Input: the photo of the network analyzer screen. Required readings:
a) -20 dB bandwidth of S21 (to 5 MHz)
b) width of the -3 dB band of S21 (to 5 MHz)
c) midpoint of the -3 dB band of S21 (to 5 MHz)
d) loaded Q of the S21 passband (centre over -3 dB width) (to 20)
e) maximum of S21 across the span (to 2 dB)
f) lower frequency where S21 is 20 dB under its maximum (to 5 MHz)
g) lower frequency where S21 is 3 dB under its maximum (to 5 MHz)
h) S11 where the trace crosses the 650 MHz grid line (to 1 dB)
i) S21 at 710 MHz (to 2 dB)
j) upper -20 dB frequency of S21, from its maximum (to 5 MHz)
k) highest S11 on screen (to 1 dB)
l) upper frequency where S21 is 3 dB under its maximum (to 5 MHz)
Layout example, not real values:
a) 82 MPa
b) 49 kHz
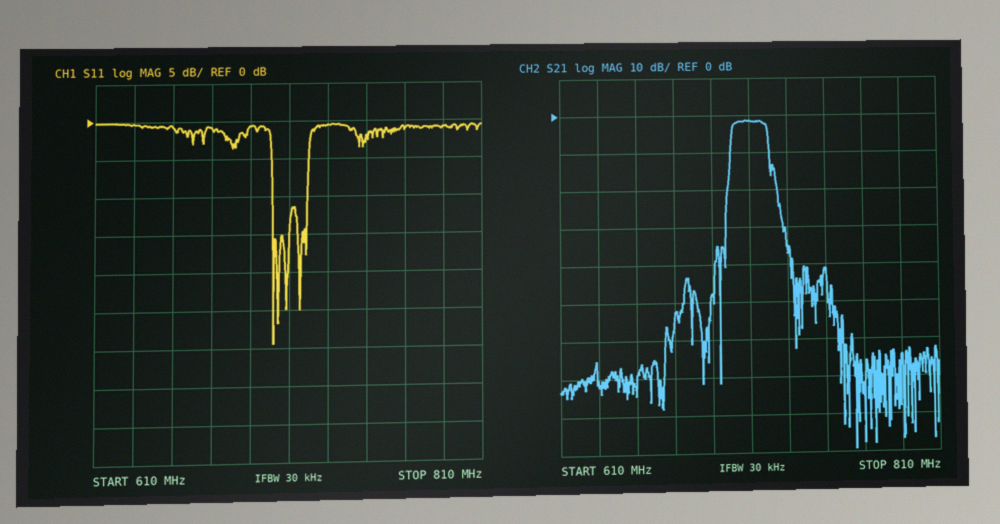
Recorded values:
a) 25 MHz
b) 20 MHz
c) 710 MHz
d) 40
e) -2 dB
f) 700 MHz
g) 700 MHz
h) -1 dB
i) -2 dB
j) 725 MHz
k) 0 dB
l) 720 MHz
